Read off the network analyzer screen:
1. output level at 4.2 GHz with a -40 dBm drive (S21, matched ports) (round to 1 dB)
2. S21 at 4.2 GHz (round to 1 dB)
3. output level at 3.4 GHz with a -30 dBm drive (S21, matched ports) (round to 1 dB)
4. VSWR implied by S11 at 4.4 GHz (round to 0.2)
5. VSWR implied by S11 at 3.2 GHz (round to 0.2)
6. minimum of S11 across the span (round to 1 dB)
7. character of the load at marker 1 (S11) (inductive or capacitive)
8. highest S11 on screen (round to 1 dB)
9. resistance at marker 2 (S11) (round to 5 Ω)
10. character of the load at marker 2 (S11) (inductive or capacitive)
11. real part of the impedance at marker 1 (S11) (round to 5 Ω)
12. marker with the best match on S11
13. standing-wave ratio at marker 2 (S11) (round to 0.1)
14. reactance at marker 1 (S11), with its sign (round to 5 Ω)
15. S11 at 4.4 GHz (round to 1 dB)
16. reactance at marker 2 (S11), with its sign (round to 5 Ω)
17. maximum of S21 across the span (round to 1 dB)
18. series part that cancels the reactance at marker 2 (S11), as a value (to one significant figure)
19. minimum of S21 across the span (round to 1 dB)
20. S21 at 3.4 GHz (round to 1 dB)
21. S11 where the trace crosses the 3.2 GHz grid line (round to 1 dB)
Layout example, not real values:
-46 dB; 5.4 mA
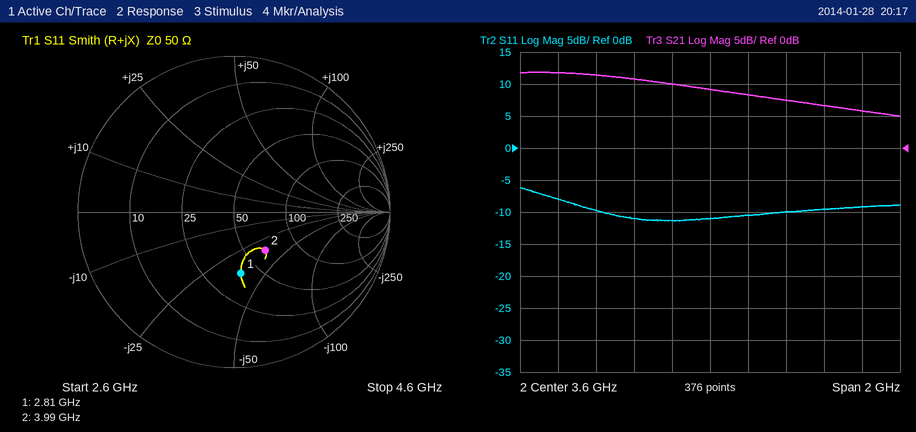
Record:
-33 dBm; 7 dB; -20 dBm; 2.0; 1.8; -11 dB; capacitive; -6 dB; 65 Ω; capacitive; 40 Ω; marker 2; 1.9; -35 Ω; -9 dB; -35 Ω; 12 dB; 1 nH; 5 dB; 10 dB; -11 dB
